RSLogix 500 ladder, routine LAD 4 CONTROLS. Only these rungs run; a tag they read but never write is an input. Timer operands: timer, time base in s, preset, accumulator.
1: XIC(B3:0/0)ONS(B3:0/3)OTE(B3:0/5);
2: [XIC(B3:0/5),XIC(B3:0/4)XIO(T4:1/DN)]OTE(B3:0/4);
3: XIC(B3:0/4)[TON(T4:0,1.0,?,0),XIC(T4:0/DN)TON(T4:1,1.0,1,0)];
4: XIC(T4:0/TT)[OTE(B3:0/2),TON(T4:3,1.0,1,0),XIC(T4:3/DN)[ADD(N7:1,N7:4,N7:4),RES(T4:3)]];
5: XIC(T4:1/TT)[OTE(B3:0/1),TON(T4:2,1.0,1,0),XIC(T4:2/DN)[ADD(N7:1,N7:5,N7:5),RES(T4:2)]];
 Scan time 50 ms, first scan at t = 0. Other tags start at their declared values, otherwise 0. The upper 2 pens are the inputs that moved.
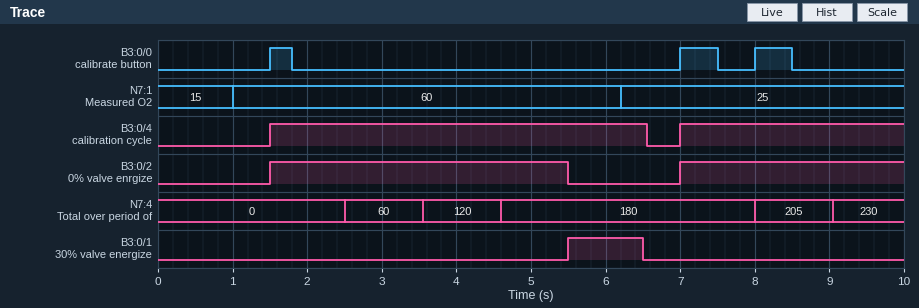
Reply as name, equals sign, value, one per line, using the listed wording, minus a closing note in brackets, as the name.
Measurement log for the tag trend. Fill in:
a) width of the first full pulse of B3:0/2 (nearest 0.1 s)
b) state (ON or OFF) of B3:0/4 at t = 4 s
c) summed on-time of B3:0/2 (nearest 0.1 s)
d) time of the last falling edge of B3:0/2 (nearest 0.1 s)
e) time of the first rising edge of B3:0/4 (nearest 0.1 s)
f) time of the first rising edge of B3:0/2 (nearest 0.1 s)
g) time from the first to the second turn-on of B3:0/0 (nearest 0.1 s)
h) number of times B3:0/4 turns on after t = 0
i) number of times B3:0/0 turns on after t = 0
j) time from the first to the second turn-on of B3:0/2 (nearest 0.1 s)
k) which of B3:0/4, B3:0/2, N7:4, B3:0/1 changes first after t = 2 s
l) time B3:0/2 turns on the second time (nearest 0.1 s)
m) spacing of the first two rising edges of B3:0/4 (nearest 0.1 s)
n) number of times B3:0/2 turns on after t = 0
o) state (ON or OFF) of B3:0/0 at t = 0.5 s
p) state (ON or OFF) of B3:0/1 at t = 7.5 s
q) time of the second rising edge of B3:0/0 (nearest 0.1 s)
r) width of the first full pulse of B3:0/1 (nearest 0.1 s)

width of the first full pulse of B3:0/2 = 4.0 s
state (ON or OFF) of B3:0/4 at t = 4 s = ON
summed on-time of B3:0/2 = 7.0 s
time of the last falling edge of B3:0/2 = 5.5 s
time of the first rising edge of B3:0/4 = 1.5 s
time of the first rising edge of B3:0/2 = 1.5 s
time from the first to the second turn-on of B3:0/0 = 5.5 s
number of times B3:0/4 turns on after t = 0 = 2
number of times B3:0/0 turns on after t = 0 = 3
time from the first to the second turn-on of B3:0/2 = 5.5 s
which of B3:0/4, B3:0/2, N7:4, B3:0/1 changes first after t = 2 s = N7:4
time B3:0/2 turns on the second time = 7.0 s
spacing of the first two rising edges of B3:0/4 = 5.5 s
number of times B3:0/2 turns on after t = 0 = 2
state (ON or OFF) of B3:0/0 at t = 0.5 s = OFF
state (ON or OFF) of B3:0/1 at t = 7.5 s = OFF
time of the second rising edge of B3:0/0 = 7.0 s
width of the first full pulse of B3:0/1 = 1.0 s
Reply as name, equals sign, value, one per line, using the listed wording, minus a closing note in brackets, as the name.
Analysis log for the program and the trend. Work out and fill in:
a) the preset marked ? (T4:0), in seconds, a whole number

the preset marked ? (T4:0), in seconds, a whole number = 4 s
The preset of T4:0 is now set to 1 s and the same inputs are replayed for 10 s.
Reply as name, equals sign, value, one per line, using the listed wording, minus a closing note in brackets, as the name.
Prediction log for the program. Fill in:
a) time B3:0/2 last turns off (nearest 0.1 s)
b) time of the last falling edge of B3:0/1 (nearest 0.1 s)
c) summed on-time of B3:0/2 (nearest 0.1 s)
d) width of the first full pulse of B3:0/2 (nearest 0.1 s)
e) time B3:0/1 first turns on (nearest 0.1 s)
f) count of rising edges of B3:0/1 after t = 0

time B3:0/2 last turns off = 8.0 s
time of the last falling edge of B3:0/1 = 9.0 s
summed on-time of B3:0/2 = 2.0 s
width of the first full pulse of B3:0/2 = 1.0 s
time B3:0/1 first turns on = 2.5 s
count of rising edges of B3:0/1 after t = 0 = 2
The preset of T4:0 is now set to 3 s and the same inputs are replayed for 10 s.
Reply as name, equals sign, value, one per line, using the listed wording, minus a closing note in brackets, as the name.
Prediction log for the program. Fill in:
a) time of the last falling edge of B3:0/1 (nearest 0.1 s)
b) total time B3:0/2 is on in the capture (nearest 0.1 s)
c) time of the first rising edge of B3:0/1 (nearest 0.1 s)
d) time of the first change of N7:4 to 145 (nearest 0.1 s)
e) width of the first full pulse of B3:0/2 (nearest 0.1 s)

time of the last falling edge of B3:0/1 = 5.5 s
total time B3:0/2 is on in the capture = 6.0 s
time of the first rising edge of B3:0/1 = 4.5 s
time of the first change of N7:4 to 145 = 8.0 s
width of the first full pulse of B3:0/2 = 3.0 s
